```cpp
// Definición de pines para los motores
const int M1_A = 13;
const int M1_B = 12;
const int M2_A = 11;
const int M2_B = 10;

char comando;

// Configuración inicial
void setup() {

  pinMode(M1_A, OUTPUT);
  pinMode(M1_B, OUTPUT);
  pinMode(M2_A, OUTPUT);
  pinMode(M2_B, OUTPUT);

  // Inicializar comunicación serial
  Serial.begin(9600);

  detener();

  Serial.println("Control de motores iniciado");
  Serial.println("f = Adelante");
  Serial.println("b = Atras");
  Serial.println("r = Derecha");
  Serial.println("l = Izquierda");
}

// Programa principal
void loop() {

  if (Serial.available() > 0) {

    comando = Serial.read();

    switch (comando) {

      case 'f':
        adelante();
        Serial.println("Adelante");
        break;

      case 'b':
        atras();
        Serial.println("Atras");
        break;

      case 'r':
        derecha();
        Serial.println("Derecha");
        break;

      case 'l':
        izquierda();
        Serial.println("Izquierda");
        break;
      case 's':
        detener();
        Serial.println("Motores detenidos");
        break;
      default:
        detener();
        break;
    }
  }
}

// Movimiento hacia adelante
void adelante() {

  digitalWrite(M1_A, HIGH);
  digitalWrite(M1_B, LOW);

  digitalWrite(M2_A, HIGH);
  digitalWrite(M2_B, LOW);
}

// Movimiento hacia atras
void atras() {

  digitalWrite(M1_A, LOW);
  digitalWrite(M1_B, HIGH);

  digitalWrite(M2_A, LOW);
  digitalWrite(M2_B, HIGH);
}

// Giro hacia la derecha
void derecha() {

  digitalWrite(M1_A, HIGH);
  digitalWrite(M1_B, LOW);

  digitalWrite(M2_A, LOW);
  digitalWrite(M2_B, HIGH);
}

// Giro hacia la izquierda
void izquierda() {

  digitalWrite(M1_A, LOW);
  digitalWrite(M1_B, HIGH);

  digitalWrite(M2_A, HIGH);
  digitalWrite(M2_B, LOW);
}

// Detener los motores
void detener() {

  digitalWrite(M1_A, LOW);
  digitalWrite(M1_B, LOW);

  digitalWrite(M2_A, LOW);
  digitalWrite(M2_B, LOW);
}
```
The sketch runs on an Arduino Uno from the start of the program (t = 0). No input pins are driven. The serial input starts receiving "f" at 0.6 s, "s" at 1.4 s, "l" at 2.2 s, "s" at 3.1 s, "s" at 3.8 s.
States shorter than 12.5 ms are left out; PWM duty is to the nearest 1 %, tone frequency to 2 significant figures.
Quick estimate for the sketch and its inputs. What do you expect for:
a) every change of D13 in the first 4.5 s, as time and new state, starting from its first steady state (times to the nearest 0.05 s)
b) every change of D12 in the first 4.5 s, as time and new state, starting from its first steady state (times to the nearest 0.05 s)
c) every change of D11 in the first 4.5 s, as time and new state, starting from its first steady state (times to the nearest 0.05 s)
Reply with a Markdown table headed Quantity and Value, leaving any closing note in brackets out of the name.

| Quantity | Value |
|---|---|
| every change of D13 in the first 4.5 s, as time and new state, starting from its first steady state | 0 s low; 0.6 s high; 1.4 s low |
| every change of D12 in the first 4.5 s, as time and new state, starting from its first steady state | 0 s low; 2.2 s high; 3.1 s low |
| every change of D11 in the first 4.5 s, as time and new state, starting from its first steady state | 0 s low; 0.6 s high; 1.4 s low; 2.2 s high; 3.1 s low |
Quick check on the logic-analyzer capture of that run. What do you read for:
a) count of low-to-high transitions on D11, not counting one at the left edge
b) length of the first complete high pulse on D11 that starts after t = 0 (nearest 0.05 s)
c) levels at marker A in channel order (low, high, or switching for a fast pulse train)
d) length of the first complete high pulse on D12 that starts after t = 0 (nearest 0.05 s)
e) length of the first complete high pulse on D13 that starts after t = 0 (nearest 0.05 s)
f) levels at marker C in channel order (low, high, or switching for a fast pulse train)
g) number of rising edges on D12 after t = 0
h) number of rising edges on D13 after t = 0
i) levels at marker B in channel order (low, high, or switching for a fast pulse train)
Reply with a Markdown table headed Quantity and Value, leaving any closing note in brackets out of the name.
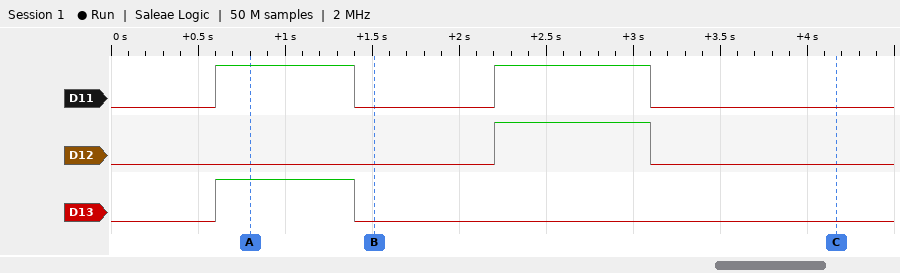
| Quantity | Value |
|---|---|
| count of low-to-high transitions on D11, not counting one at the left edge | 2 |
| length of the first complete high pulse on D11 that starts after t = 0 | 0.80 s |
| levels at marker A in channel order | D11 high, D12 low, D13 high |
| length of the first complete high pulse on D12 that starts after t = 0 | 0.90 s |
| length of the first complete high pulse on D13 that starts after t = 0 | 0.80 s |
| levels at marker C in channel order | D11 low, D12 low, D13 low |
| number of rising edges on D12 after t = 0 | 1 |
| number of rising edges on D13 after t = 0 | 1 |
| levels at marker B in channel order | D11 low, D12 low, D13 low |
